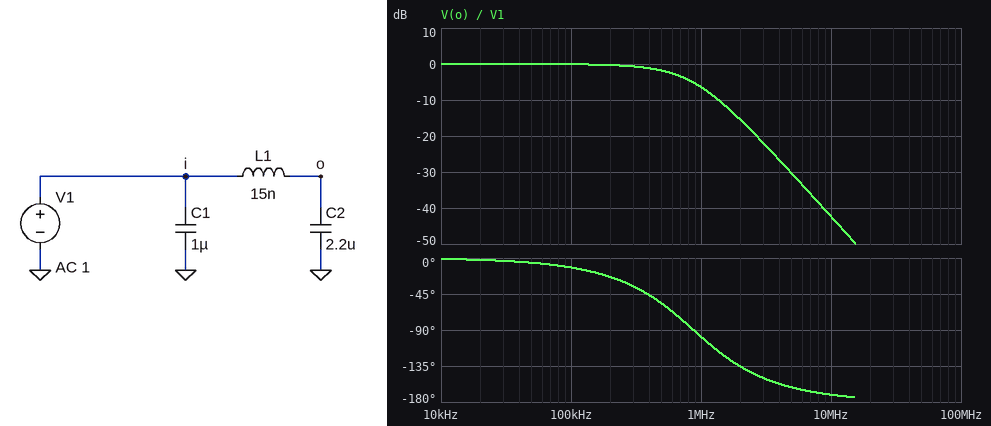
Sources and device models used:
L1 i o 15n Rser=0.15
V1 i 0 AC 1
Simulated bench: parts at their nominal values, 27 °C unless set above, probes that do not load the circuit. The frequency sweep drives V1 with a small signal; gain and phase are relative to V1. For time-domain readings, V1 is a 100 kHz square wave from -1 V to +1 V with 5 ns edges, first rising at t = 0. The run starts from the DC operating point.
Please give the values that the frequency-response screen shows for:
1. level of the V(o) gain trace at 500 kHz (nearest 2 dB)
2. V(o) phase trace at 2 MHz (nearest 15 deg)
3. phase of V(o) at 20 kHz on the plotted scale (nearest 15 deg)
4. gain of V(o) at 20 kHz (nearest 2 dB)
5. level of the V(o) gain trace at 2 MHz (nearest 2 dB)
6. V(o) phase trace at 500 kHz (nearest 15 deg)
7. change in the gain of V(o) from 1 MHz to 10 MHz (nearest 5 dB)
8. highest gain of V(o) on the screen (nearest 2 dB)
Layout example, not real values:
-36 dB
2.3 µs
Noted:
-2 dB
-135 deg
0 deg
0 dB
-16 dB
-60 deg
-35 dB
0 dB
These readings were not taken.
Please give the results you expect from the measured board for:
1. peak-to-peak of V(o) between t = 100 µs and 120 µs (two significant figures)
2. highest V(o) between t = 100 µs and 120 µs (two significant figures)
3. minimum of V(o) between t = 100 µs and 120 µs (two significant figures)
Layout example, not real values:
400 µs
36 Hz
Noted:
2.0 V
1.0 V
-1.0 V
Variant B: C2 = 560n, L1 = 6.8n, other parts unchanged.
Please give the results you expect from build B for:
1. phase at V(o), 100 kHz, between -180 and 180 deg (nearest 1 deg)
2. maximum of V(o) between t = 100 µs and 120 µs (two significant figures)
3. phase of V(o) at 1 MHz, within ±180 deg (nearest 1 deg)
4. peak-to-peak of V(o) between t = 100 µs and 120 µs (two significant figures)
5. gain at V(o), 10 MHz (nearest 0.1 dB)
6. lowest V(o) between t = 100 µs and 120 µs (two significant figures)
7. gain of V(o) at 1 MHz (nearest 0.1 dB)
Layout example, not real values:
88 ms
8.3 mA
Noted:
-3 deg
1.1 V
-32 deg
2.2 V
-23.5 dB
-1.1 V
0 dB
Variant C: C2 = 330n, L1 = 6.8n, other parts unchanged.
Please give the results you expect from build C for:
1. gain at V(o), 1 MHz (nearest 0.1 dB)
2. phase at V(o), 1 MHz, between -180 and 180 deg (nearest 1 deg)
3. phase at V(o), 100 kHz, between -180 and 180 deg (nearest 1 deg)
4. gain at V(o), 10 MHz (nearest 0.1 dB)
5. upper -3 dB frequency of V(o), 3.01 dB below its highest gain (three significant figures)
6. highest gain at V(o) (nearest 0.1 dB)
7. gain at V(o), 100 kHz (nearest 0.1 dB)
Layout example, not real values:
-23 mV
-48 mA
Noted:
0.3 dB
-19 deg
-2 deg
-18.5 dB
3.90 MHz
1.0 dB
0 dB
